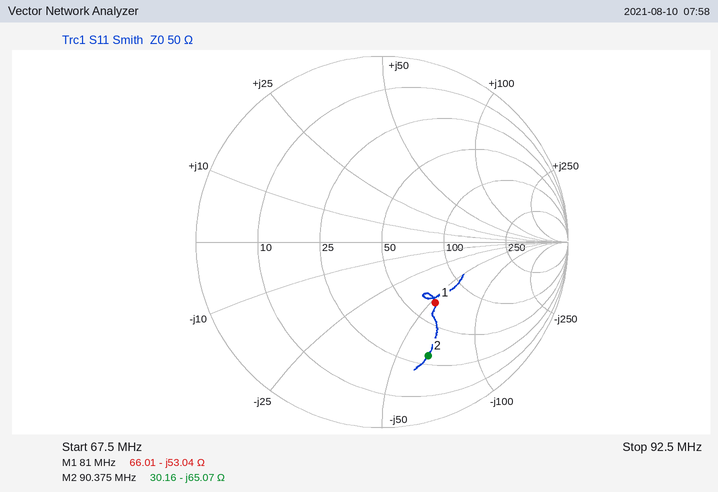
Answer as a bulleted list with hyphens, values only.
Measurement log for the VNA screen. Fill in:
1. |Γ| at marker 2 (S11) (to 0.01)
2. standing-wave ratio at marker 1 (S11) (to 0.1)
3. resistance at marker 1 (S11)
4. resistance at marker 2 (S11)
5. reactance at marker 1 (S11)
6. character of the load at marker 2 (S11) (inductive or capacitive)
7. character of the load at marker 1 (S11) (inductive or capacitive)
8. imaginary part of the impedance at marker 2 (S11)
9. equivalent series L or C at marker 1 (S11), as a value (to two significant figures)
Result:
- 0.66
- 2.5
- 66.01 Ω
- 30.16 Ω
- -53.04 Ω
- capacitive
- capacitive
- -65.07 Ω
- 37 pF
